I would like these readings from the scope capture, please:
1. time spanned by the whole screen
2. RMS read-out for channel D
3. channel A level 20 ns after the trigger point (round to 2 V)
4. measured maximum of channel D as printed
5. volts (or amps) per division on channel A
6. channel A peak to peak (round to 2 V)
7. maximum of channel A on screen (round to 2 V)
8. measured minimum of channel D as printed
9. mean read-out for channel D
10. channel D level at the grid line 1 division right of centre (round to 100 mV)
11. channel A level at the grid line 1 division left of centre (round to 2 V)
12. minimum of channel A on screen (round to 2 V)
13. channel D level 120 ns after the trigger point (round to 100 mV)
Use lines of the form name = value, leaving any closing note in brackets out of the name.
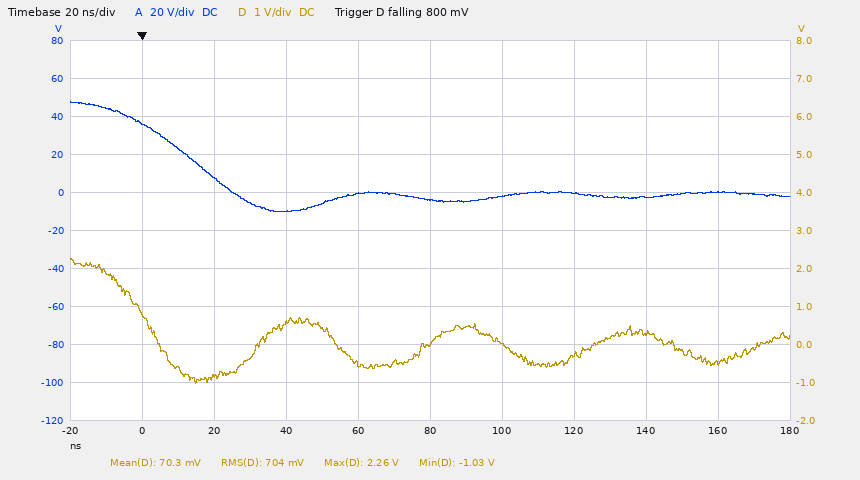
time spanned by the whole screen = 200 ns
RMS read-out for channel D = 704 mV
channel A level 20 ns after the trigger point = 8 V
measured maximum of channel D as printed = 2.26 V
volts (or amps) per division on channel A = 20 V
channel A peak to peak = 58 V
maximum of channel A on screen = 48 V
measured minimum of channel D as printed = -1.03 V
mean read-out for channel D = 70.3 mV
channel D level at the grid line 1 division right of centre = 0.0 V
channel A level at the grid line 1 division left of centre = 0 V
minimum of channel A on screen = -10 V
channel D level 120 ns after the trigger point = -300 mV
